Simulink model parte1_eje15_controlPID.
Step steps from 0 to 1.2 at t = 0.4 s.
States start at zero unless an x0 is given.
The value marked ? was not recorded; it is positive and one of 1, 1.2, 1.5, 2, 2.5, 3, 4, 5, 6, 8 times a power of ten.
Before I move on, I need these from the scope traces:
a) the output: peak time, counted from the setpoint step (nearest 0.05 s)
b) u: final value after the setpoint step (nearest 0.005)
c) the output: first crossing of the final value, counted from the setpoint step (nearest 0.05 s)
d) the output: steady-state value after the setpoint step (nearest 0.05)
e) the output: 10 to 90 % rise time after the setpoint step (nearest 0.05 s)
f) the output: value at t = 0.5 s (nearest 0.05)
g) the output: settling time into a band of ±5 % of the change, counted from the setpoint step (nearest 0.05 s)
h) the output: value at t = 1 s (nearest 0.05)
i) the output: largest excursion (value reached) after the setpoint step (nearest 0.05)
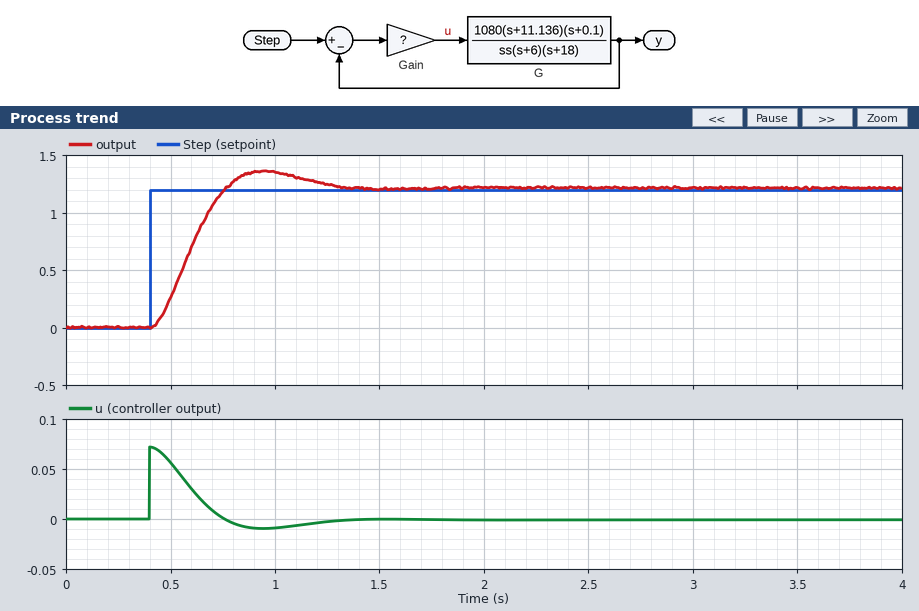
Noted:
0.55 s
0.000
0.35 s
1.20
0.25 s
0.25
0.80 s
1.35
1.35
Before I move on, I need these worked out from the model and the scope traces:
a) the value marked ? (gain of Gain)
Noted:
0.06
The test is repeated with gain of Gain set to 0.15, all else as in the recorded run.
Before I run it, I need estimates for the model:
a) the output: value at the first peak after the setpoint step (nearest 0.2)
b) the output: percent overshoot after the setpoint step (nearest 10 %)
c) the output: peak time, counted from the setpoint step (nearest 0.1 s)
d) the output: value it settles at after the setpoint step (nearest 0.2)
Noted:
1.6
30 %
0.3 s
1.2
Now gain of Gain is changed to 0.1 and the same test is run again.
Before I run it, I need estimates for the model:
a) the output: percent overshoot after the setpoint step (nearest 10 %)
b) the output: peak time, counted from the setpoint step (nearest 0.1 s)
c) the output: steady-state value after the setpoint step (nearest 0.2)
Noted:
20 %
0.4 s
1.2
